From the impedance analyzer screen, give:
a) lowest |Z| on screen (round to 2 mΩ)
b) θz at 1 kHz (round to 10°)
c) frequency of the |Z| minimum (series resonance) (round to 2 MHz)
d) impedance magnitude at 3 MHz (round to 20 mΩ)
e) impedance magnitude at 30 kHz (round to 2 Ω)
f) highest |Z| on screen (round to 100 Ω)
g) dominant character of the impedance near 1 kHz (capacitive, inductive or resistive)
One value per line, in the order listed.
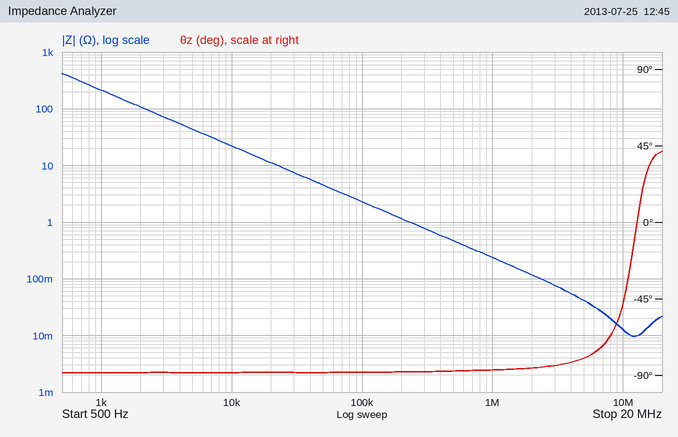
10 mΩ
-90°
12 MHz
80 mΩ
8 Ω
400 Ω
capacitive
